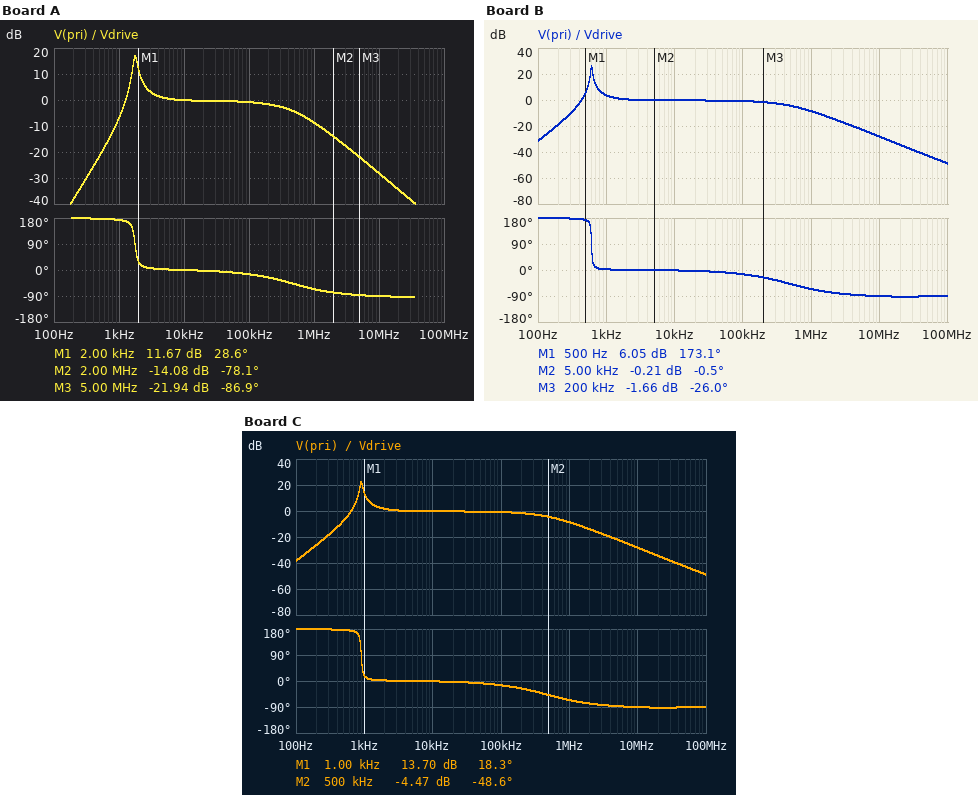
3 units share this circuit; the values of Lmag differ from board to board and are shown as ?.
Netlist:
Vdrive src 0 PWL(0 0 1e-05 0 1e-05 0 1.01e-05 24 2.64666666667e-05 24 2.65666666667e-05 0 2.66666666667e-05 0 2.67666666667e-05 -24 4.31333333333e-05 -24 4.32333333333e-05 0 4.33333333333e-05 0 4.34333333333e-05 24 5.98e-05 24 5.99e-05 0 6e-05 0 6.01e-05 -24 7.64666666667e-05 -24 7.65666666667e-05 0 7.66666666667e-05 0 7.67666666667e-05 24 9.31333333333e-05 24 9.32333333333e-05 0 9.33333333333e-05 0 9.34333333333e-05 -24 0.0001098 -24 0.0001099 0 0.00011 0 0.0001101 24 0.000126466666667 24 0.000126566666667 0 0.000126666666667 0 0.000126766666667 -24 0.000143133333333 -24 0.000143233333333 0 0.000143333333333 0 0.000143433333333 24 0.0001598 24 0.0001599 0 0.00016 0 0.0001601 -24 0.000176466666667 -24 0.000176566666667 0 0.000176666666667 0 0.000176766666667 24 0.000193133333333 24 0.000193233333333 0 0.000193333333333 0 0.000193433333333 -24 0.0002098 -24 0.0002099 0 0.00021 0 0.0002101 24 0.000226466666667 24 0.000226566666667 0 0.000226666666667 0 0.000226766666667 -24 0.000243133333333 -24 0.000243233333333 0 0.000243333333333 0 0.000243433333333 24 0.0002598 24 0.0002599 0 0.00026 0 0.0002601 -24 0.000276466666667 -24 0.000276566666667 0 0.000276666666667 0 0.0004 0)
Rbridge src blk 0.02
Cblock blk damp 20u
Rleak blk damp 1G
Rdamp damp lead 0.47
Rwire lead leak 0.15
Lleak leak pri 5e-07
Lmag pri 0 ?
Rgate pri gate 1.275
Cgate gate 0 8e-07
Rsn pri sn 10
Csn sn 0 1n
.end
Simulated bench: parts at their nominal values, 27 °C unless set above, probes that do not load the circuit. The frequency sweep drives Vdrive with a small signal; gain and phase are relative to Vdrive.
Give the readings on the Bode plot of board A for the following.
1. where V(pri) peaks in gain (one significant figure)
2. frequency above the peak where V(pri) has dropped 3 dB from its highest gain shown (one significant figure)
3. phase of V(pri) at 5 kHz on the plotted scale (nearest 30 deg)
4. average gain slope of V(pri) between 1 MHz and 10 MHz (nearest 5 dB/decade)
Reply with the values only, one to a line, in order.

2 kHz
2 kHz
0 deg
-20 dB/decade
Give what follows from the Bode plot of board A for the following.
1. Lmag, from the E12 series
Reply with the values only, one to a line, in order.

390 µH
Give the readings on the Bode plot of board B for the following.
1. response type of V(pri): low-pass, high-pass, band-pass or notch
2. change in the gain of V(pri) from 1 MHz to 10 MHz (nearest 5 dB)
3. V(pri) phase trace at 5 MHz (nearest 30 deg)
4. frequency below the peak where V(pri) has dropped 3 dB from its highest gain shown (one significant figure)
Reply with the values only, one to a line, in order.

band-pass
-20 dB
-90 deg
600 Hz
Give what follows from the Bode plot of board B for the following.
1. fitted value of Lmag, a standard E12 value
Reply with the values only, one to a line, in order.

3.3 mH
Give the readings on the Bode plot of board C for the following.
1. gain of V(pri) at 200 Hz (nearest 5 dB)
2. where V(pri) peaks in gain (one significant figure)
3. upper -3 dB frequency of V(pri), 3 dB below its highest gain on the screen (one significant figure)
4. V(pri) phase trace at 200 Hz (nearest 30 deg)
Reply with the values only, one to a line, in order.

-25 dB
900 Hz
900 Hz
180 deg
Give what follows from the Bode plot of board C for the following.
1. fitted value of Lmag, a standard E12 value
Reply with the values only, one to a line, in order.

1.5 mH
